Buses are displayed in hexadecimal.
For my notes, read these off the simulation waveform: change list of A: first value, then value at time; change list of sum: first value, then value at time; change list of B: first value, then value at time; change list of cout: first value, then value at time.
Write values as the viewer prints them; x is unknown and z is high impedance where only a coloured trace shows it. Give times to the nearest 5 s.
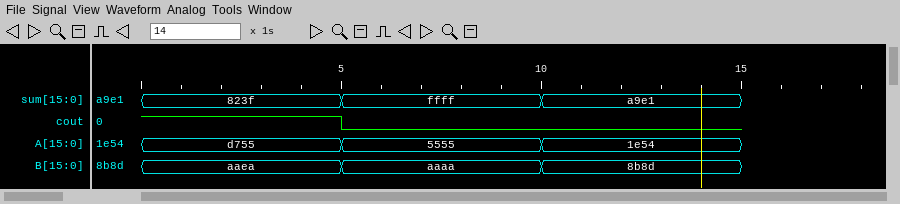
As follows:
d755, 5555 at 5 s, 1e54 at 10 s
823f, ffff at 5 s, a9e1 at 10 s
aaea, aaaa at 5 s, 8b8d at 10 s
1, 0 at 5 s
